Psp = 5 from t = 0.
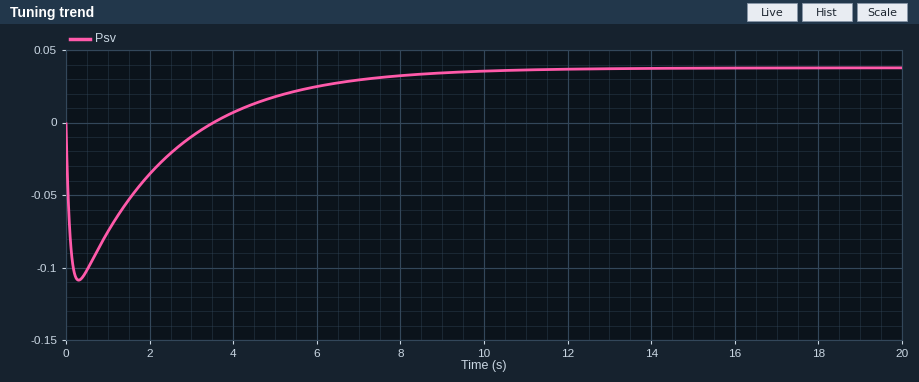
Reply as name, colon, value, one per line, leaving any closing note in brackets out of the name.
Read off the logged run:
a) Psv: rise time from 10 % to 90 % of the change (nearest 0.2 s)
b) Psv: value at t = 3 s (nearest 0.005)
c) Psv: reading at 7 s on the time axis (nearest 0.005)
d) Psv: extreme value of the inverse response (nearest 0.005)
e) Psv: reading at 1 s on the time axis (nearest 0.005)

Psv: rise time from 10 % to 90 % of the change: 5.0 s
Psv: value at t = 3 s: -0.010
Psv: reading at 7 s on the time axis: 0.030
Psv: extreme value of the inverse response: -0.110
Psv: reading at 1 s on the time axis: -0.075
